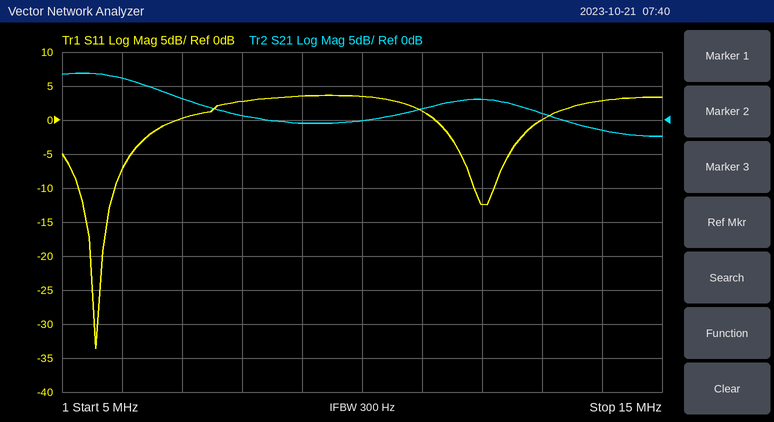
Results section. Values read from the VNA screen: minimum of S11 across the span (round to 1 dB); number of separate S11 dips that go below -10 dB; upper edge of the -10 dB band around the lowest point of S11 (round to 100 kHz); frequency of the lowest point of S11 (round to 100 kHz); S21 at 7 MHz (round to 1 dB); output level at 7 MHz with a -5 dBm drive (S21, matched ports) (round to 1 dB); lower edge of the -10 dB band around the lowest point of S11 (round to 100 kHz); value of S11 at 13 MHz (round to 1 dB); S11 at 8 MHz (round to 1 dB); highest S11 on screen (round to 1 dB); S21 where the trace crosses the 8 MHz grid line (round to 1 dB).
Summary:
-34 dB
2
5.9 MHz
5.6 MHz
3 dB
-2 dBm
5.3 MHz
0 dB
3 dB
4 dB
1 dB
